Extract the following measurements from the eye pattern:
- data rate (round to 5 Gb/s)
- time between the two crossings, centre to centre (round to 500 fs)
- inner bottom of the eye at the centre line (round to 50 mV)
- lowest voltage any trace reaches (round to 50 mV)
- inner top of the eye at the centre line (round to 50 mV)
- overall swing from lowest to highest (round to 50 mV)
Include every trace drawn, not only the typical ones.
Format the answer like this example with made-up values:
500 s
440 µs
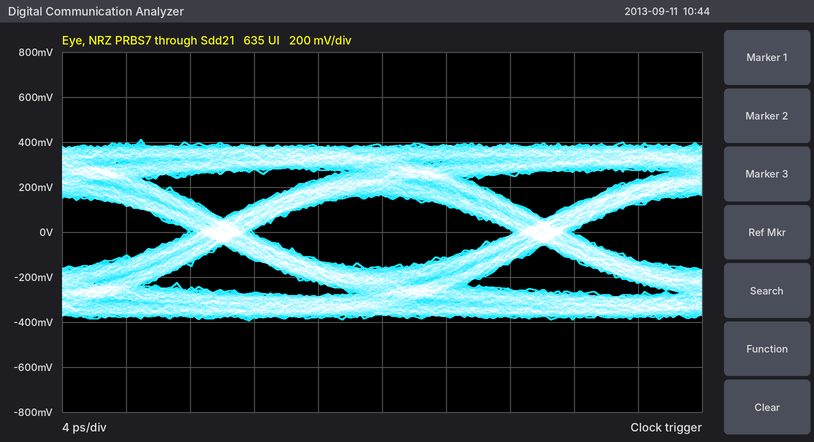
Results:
50 Gb/s
20.0 ps
-150 mV
-400 mV
150 mV
800 mV
